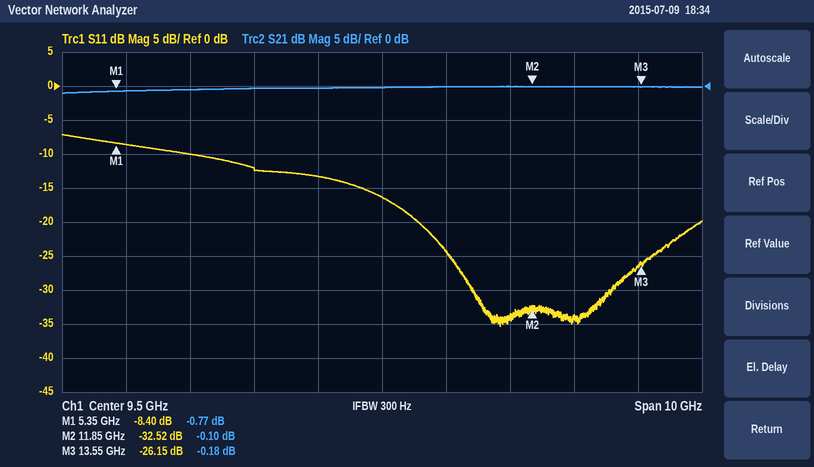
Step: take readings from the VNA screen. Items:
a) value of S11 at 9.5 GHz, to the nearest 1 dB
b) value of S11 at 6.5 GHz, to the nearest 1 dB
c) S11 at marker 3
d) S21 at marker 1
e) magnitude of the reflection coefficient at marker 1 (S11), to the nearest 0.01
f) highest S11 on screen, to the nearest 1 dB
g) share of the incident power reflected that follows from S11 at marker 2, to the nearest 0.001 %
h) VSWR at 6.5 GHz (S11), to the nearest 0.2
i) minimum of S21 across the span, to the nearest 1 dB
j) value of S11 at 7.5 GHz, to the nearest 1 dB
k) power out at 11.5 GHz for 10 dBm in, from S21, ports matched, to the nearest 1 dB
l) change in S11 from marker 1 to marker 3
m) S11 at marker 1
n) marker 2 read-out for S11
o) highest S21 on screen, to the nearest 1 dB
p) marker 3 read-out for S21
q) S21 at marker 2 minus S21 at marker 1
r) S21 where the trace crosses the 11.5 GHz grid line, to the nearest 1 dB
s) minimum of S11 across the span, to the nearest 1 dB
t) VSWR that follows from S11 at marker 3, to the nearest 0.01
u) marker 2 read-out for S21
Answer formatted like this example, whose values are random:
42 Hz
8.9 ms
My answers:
-16 dB
-10 dB
-26.15 dB
-0.77 dB
0.38
-7 dB
0.056 %
2.0
-1 dB
-12 dB
10 dBm
-17.75 dB
-8.40 dB
-32.52 dB
0 dB
-0.18 dB
0.67 dB
0 dB
-35 dB
1.10
-0.10 dB
